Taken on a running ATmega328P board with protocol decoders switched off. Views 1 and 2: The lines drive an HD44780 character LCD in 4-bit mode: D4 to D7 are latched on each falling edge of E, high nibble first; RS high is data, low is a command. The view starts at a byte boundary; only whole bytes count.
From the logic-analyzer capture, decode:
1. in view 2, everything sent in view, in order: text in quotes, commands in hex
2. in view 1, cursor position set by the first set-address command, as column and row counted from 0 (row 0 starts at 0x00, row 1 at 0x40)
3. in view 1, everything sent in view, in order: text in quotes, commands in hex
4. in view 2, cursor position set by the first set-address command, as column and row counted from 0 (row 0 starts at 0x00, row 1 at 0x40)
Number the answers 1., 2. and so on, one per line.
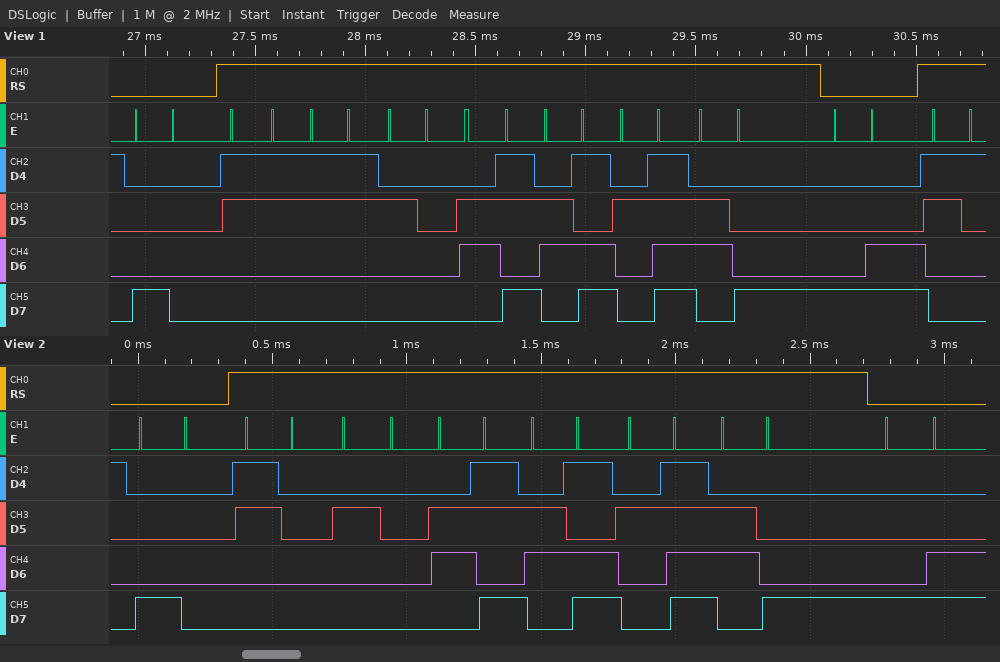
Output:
1. 0x80 "0 km/h" 0x8C
2. column 0, row 0
3. 0x80 "33 km/h" 0x8C "1"
4. column 0, row 0
